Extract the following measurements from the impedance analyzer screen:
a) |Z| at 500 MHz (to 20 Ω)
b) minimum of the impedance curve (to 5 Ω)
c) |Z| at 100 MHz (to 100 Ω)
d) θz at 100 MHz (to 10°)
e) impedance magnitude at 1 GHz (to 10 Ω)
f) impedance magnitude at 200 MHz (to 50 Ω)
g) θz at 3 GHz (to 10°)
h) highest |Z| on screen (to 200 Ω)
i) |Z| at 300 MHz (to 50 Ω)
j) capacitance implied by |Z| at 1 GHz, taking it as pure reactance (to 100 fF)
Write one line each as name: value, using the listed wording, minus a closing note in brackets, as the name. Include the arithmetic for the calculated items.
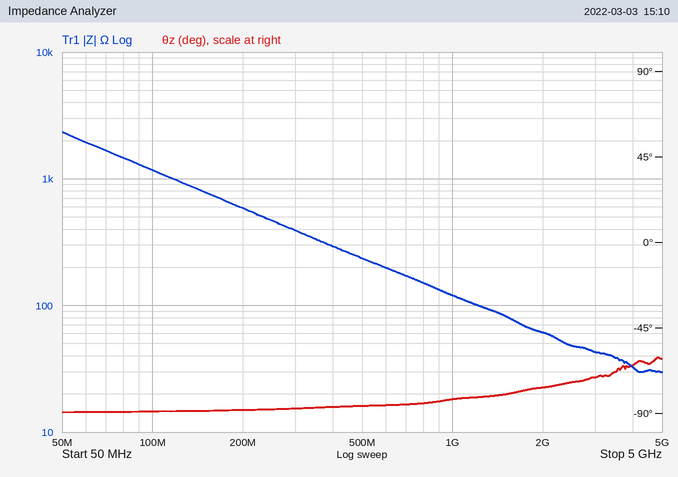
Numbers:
|Z| at 500 MHz: 240 Ω
minimum of the impedance curve: 30 Ω
|Z| at 100 MHz: 1.2 kΩ
θz at 100 MHz: -90°
impedance magnitude at 1 GHz: 120 Ω
impedance magnitude at 200 MHz: 600 Ω
θz at 3 GHz: -70°
highest |Z| on screen: 2.4 kΩ
|Z| at 300 MHz: 400 Ω
capacitance implied by |Z| at 1 GHz, taking it as pure reactance: C = 1/(2π × 1 GHz × 120 Ω) ≈ 1.3 pF
